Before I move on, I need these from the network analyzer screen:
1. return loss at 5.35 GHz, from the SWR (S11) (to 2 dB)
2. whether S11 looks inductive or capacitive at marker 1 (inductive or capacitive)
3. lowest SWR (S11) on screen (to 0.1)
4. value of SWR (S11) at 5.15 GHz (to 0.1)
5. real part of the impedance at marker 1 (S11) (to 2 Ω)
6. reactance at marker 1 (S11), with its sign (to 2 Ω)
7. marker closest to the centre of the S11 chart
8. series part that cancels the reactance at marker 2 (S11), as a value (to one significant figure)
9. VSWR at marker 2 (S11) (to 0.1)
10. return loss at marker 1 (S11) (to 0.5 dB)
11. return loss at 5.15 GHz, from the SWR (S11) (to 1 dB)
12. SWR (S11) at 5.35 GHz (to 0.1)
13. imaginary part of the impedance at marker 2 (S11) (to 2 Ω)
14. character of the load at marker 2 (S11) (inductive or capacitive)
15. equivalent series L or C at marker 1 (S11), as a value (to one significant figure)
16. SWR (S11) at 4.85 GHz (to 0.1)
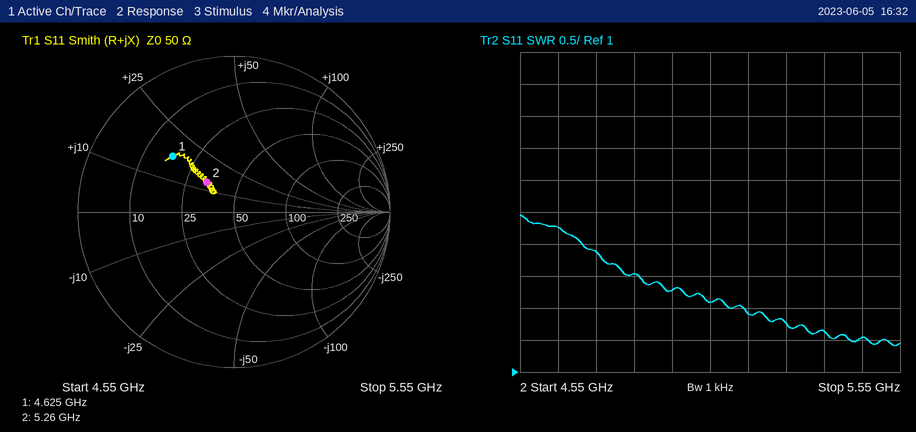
12 dB
inductive
1.4
1.9
18 Ω
+18 Ω
marker 2
2 pF
1.7
5.5 dB
10 dB
1.6
+14 Ω
inductive
600 pH
2.5
